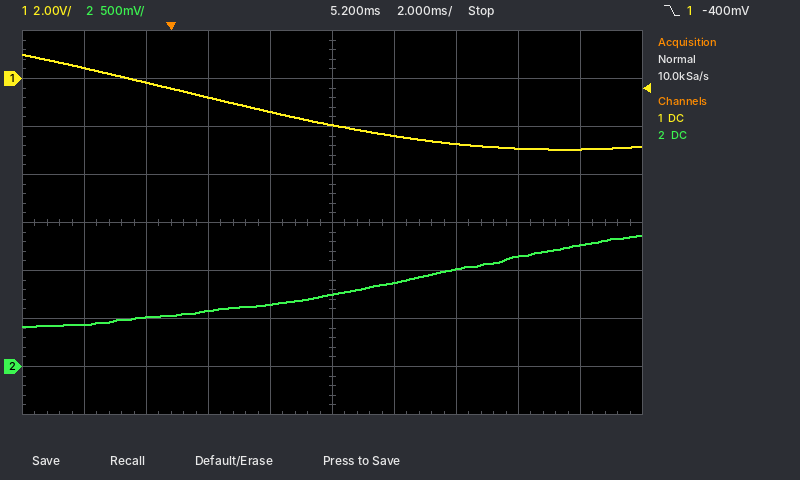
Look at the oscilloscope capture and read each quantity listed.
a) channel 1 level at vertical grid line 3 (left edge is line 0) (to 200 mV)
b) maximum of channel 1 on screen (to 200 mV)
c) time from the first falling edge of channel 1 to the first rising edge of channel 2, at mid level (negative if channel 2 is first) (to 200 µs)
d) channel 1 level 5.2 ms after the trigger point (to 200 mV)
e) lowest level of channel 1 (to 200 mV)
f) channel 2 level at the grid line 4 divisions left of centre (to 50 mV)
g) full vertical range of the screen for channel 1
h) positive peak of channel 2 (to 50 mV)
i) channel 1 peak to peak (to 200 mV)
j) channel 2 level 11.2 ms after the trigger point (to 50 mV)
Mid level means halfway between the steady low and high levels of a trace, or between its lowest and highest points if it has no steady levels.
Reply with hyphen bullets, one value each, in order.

- -800 mV
- 1.0 V
- +5.6 ms
- -2.0 V
- -3.0 V
- 450 mV
- 16 V
- 1.35 V
- 4.0 V
- 1.15 V
